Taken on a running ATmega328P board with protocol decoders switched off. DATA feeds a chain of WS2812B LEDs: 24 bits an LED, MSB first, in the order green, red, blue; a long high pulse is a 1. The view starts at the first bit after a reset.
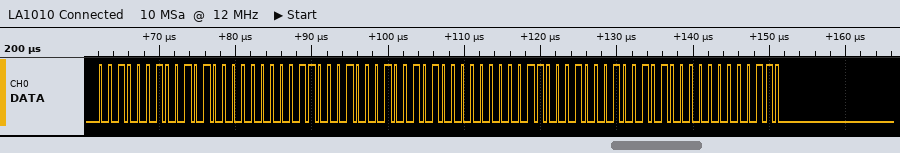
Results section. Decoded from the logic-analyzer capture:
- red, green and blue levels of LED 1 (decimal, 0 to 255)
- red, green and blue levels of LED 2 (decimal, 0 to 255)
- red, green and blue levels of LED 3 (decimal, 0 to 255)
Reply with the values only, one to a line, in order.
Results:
80, 34, 6
80, 34, 6
80, 34, 6
